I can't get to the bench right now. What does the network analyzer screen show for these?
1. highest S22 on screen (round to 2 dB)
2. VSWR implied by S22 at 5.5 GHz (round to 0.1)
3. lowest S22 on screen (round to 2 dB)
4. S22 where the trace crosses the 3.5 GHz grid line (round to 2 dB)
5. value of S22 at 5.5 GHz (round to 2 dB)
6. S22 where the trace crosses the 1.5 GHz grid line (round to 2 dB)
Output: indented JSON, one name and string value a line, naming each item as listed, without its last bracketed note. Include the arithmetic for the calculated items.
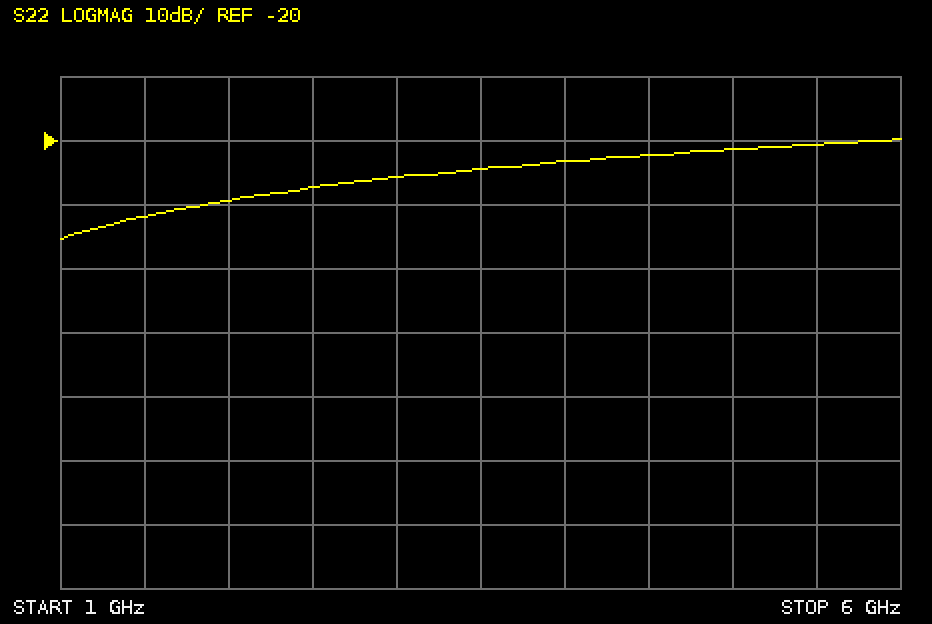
{
  "highest S22 on screen": "-20 dB",
  "VSWR implied by S22 at 5.5 GHz": "|Γ| = 10^(-20/20) = 0.1000; VSWR = (1 + 0.1000)/(1 − 0.1000) ≈ 1.2",
  "lowest S22 on screen": "-36 dB",
  "S22 where the trace crosses the 3.5 GHz grid line": "-24 dB",
  "value of S22 at 5.5 GHz": "-20 dB",
  "S22 where the trace crosses the 1.5 GHz grid line": "-32 dB"
}
